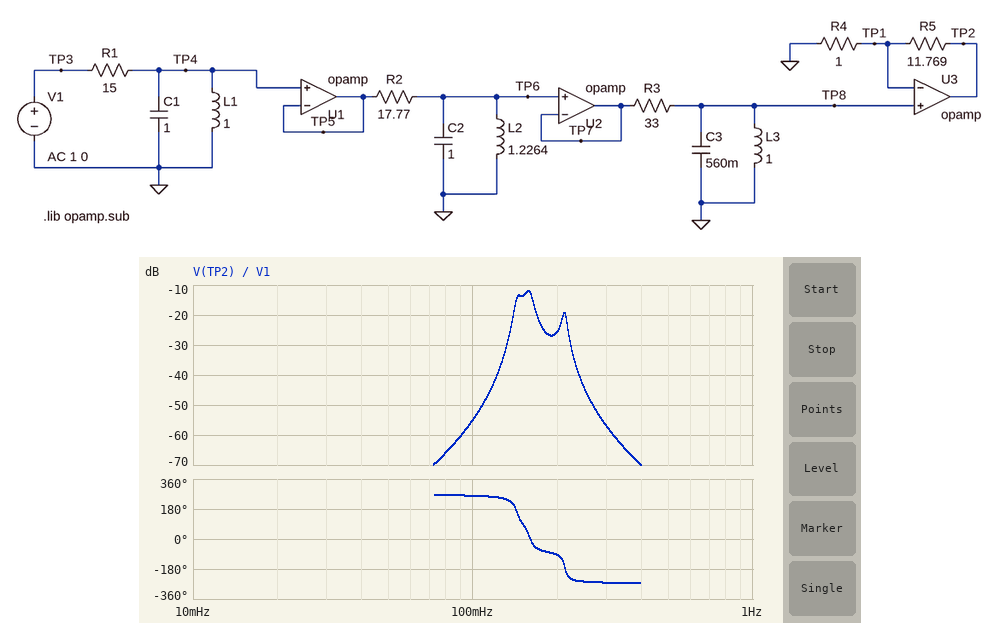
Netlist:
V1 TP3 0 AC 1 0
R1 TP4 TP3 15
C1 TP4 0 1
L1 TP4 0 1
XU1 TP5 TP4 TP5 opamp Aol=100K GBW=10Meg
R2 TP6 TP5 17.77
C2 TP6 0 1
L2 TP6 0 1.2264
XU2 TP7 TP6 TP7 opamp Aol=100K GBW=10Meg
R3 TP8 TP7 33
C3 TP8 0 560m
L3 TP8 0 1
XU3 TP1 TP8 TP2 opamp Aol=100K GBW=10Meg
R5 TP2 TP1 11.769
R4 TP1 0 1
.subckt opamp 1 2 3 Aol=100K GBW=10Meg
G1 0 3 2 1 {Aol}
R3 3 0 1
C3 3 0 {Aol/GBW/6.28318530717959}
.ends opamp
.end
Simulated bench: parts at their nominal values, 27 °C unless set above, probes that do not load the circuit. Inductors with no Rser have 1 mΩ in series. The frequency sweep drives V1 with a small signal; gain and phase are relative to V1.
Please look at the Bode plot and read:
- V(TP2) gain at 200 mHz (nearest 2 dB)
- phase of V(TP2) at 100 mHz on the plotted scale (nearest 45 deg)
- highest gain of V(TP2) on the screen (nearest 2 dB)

-26 dB
270 deg
-12 dB
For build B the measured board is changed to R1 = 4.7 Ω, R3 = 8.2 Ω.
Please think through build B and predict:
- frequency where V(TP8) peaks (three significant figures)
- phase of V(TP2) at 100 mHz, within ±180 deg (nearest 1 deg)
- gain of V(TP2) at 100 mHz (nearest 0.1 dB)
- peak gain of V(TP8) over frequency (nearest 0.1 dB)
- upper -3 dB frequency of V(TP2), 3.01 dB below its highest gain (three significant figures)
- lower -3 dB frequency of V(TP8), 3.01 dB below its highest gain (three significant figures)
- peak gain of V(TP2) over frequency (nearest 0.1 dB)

145 mHz
-113 deg
-32.9 dB
-16.8 dB
152 mHz
141 mHz
5.3 dB
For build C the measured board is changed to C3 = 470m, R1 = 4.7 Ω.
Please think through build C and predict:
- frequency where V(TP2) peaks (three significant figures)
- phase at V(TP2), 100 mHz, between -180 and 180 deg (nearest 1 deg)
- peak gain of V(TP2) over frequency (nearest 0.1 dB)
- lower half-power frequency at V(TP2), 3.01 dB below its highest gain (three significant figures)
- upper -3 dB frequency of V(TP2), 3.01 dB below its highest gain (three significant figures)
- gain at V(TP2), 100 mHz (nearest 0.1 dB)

145 mHz
-109 deg
-7.7 dB
141 mHz
152 mHz
-45.4 dB
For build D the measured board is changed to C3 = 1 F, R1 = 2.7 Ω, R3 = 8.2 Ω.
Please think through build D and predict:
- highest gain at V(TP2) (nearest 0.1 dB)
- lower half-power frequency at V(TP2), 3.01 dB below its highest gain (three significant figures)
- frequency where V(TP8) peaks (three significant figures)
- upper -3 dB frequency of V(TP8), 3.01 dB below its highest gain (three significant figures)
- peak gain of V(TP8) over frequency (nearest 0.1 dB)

15.4 dB
141 mHz
145 mHz
156 mHz
-6.7 dB
